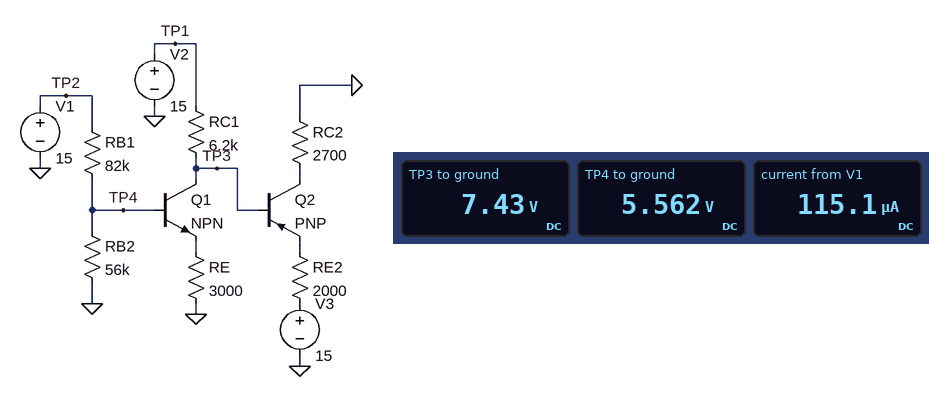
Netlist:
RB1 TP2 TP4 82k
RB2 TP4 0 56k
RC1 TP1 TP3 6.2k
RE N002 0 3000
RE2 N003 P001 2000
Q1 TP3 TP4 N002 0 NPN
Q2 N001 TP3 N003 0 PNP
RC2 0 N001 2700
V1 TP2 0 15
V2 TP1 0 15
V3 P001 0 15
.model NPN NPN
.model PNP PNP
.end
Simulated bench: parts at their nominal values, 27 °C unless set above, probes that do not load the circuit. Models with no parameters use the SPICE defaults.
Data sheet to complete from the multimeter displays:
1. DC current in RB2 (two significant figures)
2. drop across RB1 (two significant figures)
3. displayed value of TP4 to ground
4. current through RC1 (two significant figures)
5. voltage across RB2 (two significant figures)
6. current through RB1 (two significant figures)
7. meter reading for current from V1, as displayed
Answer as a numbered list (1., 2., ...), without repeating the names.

1. 99 µA
2. 9.4 V
3. 5.562 V
4. 1.2 mA
5. 5.6 V
6. 120 µA
7. 115.1 µA
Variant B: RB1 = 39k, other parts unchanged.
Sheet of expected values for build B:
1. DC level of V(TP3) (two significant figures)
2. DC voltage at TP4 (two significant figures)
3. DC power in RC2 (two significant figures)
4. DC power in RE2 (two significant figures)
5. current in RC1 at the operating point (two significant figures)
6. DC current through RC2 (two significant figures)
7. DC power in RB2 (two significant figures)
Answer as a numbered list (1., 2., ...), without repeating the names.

1. 6.8 V
2. 7.5 V
3. 21 mW
4. 27 mW
5. 1.3 mA
6. 2.8 mA
7. 1.0 mW
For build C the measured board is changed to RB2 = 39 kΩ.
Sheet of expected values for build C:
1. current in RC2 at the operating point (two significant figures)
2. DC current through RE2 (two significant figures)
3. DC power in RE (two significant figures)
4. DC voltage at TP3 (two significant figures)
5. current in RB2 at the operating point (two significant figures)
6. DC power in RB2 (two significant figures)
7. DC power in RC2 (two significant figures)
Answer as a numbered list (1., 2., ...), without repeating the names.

1. 3.1 mA
2. 3.2 mA
3. 4.6 mW
4. 7.8 V
5. 120 µA
6. 520 µW
7. 27 mW
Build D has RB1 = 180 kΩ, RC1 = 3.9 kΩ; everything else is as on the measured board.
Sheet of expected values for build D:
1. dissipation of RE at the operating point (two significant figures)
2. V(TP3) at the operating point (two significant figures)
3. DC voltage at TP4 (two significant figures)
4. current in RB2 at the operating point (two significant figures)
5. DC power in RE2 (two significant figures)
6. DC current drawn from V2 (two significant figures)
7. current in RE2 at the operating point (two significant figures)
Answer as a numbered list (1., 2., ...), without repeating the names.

1. 2.0 mW
2. 12 V
3. 3.2 V
4. 57 µA
5. 2.7 mW
6. 800 µA
7. 1.2 mA
